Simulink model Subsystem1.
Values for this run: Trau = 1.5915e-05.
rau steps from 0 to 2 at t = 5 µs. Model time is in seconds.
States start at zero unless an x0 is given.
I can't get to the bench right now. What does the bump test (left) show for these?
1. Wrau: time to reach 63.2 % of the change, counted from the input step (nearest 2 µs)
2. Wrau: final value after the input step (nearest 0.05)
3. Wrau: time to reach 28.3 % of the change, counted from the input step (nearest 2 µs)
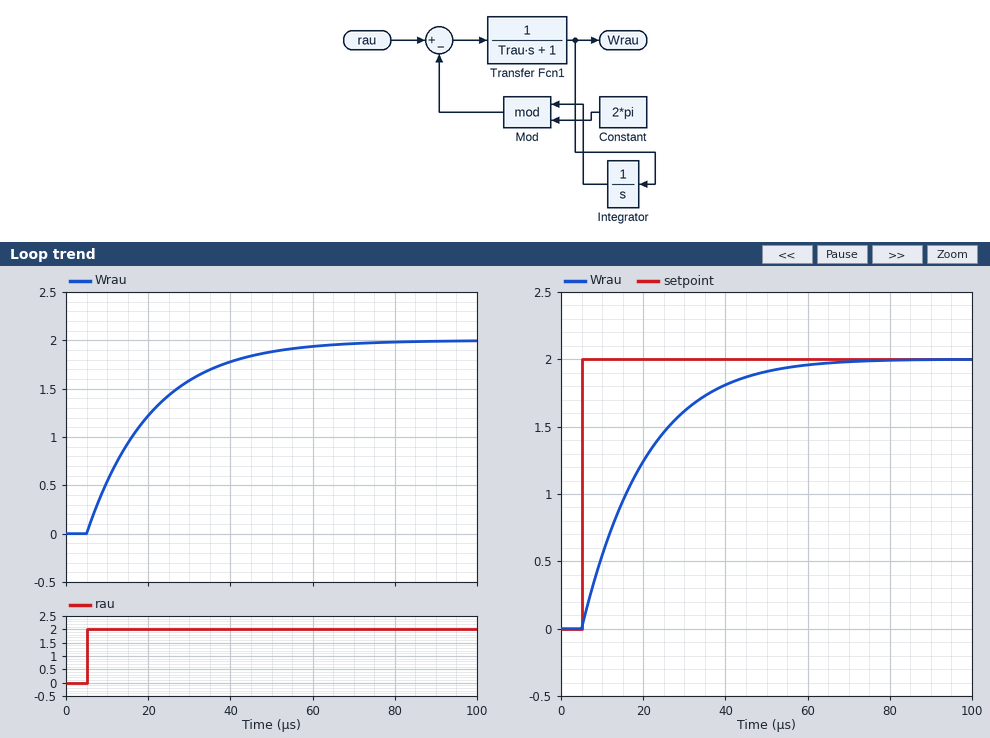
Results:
16 µs
2.00
6 µs
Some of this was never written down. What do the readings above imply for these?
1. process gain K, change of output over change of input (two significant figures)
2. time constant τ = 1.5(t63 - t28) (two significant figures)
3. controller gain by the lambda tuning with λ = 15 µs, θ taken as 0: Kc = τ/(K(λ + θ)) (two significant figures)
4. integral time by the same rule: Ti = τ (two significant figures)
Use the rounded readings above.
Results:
1.0
15 µs
1.0
15 µs
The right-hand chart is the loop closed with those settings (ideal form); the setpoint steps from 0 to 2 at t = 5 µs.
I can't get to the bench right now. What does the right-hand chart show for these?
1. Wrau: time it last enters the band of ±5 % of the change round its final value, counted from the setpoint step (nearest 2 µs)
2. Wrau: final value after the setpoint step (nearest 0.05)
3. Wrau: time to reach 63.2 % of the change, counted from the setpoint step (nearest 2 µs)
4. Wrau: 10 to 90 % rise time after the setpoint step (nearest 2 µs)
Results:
44 µs
2.00
16 µs
32 µs
